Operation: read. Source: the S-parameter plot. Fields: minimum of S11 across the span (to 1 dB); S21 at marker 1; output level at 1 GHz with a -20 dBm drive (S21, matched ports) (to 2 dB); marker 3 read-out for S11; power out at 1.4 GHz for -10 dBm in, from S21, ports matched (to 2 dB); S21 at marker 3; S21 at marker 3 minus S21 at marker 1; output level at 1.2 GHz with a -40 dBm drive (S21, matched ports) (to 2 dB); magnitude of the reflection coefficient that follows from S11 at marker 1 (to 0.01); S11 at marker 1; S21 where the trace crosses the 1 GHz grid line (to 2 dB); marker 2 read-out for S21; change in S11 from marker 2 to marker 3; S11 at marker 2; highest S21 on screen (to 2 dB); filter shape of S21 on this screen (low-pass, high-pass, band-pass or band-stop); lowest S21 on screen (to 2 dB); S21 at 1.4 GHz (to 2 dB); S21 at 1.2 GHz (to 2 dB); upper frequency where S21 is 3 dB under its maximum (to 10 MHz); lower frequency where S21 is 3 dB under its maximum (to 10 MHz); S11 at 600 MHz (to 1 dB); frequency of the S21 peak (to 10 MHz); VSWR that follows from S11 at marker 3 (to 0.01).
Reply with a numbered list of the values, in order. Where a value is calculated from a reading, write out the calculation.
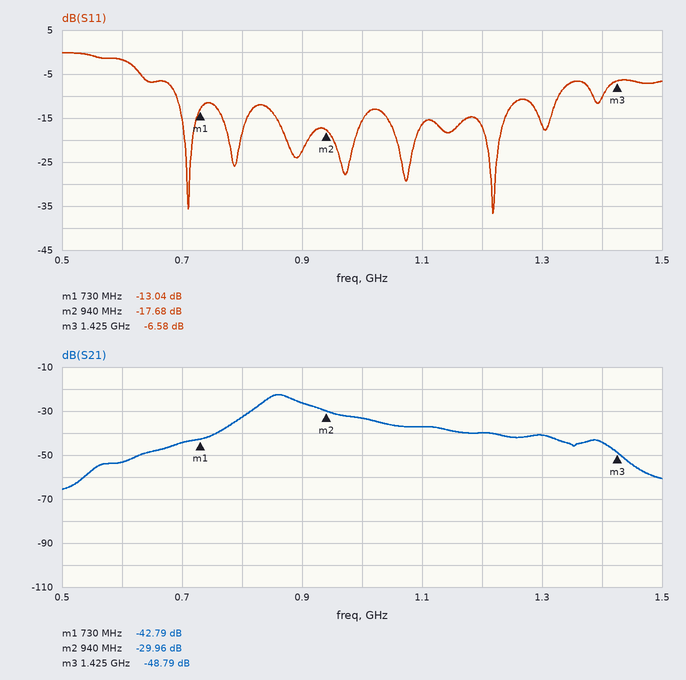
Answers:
1. -37 dB
2. -42.79 dB
3. -20 dBm + (-34 dB) = -54 dBm
4. -6.58 dB
5. -10 dBm + (-44 dB) = -54 dBm
6. -48.79 dB
7. -48.79 − (-42.79) = -6.00 dB
8. -40 dBm + (-40 dB) = -80 dBm
9. 10^(-13.04/20) ≈ 0.22
10. -13.04 dB
11. -34 dB
12. -29.96 dB
13. -6.58 − (-17.68) = 11.10 dB
14. -17.68 dB
15. -22 dB
16. band-pass
17. -66 dB
18. -44 dB
19. -40 dB
20. 890 MHz
21. 840 MHz
22. -2 dB
23. 860 MHz
24. (1 + 0.4688)/(1 − 0.4688) ≈ 2.77
